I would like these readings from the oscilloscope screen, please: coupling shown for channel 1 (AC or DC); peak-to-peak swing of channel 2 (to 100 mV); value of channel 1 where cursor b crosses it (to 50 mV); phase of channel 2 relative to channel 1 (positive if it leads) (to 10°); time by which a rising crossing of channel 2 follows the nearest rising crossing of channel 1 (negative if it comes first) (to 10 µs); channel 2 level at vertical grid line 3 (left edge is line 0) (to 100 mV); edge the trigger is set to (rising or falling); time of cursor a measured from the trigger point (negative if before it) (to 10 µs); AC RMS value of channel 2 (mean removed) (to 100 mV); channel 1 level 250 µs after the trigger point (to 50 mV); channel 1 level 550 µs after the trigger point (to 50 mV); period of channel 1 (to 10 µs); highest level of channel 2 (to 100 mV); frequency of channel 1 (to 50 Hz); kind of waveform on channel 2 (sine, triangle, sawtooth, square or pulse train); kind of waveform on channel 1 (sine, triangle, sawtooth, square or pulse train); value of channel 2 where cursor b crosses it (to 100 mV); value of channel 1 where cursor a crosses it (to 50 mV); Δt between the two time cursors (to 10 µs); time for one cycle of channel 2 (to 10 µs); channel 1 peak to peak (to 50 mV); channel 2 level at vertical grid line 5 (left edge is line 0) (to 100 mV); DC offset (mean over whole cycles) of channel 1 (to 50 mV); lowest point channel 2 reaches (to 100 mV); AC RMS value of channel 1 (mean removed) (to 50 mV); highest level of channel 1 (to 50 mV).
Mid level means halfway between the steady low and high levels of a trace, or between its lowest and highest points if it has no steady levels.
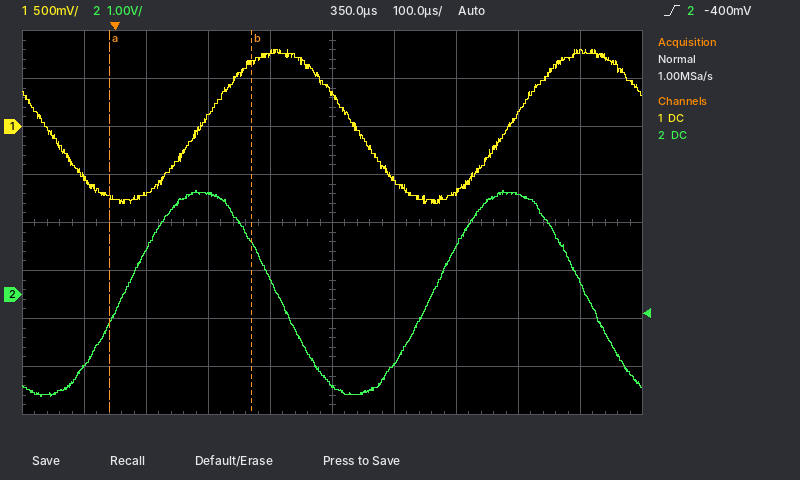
DC
4.3 V
650 mV
+90°
-120 µs
2.1 V
rising
-10 µs
1.5 V
750 mV
-700 mV
500 µs
2.2 V
2.00 kHz
sine
sine
1.1 V
-750 mV
230 µs
500 µs
1.60 V
-1.9 V
0 mV
-2.1 V
550 mV
800 mV
